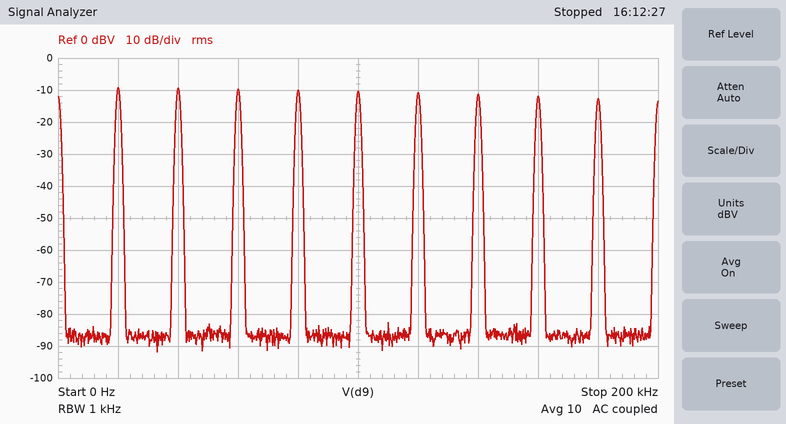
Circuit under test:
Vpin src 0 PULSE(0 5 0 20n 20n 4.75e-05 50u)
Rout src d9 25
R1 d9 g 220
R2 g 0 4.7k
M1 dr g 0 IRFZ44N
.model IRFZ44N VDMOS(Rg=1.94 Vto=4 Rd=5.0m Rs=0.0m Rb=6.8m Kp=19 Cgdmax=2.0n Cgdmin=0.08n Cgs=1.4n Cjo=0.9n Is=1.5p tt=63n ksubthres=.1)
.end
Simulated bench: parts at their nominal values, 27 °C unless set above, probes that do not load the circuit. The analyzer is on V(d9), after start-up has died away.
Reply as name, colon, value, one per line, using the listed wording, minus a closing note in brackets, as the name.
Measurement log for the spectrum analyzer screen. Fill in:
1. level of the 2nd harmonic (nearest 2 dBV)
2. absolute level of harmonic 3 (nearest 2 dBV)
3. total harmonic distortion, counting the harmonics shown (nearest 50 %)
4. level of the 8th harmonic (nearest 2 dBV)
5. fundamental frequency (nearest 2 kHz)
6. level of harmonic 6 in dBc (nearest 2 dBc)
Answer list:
level of the 2nd harmonic: -10 dBV
absolute level of harmonic 3: -10 dBV
total harmonic distortion, counting the harmonics shown: 250 %
level of the 8th harmonic: -12 dBV
fundamental frequency: 20 kHz
level of harmonic 6 in dBc: -2 dBc
